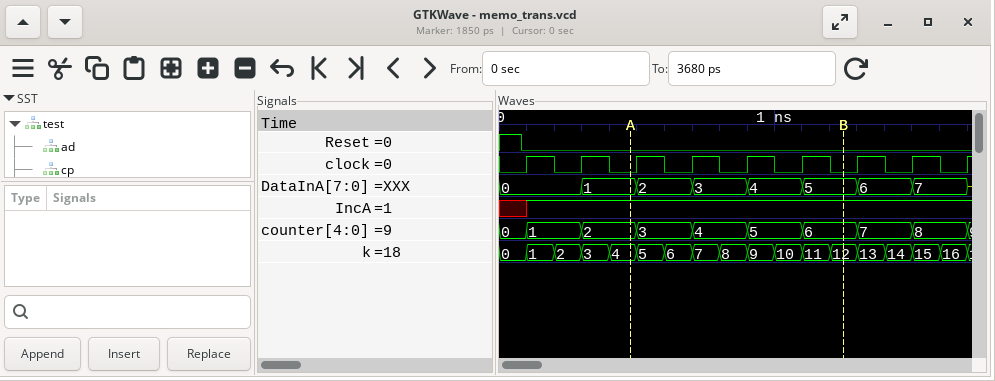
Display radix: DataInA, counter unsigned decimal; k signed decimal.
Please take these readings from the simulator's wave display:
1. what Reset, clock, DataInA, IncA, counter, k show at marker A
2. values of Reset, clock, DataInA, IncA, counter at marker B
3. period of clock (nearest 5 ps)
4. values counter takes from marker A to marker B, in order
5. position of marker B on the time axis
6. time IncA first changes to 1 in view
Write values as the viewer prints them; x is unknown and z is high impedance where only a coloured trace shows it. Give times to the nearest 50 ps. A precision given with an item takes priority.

Reset=0, clock=0, DataInA=1, IncA=1, counter=2, k=4
Reset=0, clock=0, DataInA=5, IncA=1, counter=6
200 ps
2, 3, 4, 5, 6
1250 ps
100 ps
